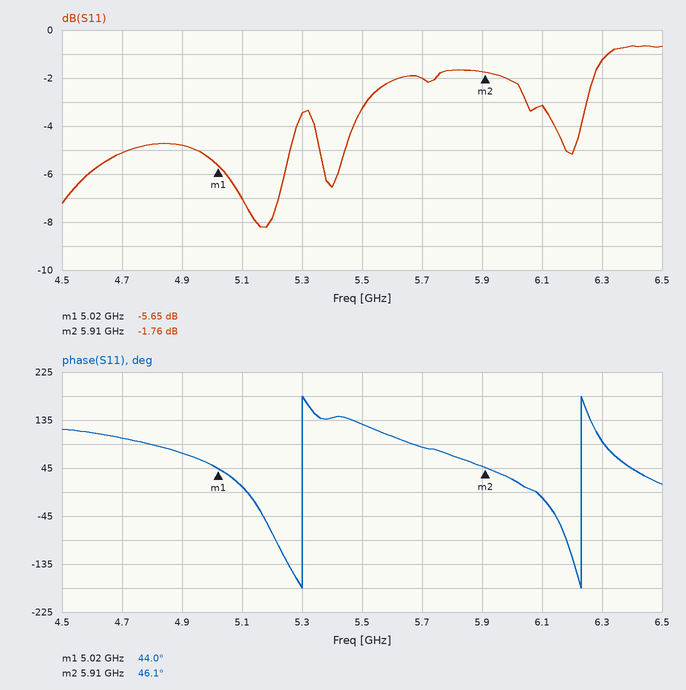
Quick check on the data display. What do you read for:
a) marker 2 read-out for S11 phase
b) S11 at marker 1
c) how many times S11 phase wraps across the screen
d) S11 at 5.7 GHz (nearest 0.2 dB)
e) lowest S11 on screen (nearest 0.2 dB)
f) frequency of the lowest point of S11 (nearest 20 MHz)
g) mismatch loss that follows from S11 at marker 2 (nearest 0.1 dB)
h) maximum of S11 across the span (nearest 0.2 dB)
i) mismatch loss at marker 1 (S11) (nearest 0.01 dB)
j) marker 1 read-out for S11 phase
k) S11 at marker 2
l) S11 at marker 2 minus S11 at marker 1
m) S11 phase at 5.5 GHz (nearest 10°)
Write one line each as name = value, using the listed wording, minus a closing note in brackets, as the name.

marker 2 read-out for S11 phase = 46.1°
S11 at marker 1 = -5.65 dB
how many times S11 phase wraps across the screen = 2
S11 at 5.7 GHz = -2.0 dB
lowest S11 on screen = -8.2 dB
frequency of the lowest point of S11 = 5.18 GHz
mismatch loss that follows from S11 at marker 2 = 4.8 dB
maximum of S11 across the span = -0.6 dB
mismatch loss at marker 1 (S11) = 1.38 dB
marker 1 read-out for S11 phase = 44.0°
S11 at marker 2 = -1.76 dB
S11 at marker 2 minus S11 at marker 1 = 3.89 dB
S11 phase at 5.5 GHz = 130°
